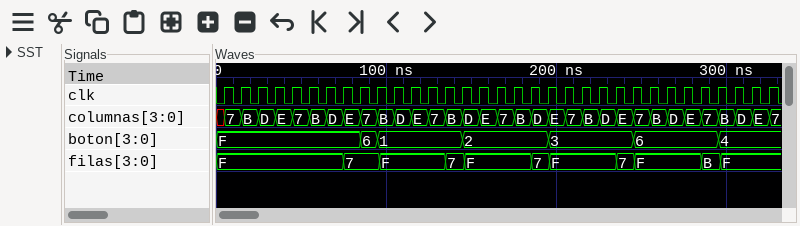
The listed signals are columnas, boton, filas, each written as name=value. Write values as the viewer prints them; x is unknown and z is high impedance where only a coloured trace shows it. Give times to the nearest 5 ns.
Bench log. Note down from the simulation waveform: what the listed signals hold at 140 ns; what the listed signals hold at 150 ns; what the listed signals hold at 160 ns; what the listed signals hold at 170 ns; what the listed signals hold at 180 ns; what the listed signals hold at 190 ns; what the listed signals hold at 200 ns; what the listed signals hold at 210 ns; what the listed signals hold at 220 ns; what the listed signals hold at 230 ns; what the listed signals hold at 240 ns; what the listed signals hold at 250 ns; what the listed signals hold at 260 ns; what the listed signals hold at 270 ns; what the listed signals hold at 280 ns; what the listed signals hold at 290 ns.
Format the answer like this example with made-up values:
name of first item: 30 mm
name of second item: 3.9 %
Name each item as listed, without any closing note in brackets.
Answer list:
what the listed signals hold at 140 ns: columnas=B, boton=1, filas=7
what the listed signals hold at 150 ns: columnas=D, boton=2, filas=F
what the listed signals hold at 160 ns: columnas=E, boton=2, filas=F
what the listed signals hold at 170 ns: columnas=7, boton=2, filas=F
what the listed signals hold at 180 ns: columnas=B, boton=2, filas=F
what the listed signals hold at 190 ns: columnas=D, boton=2, filas=7
what the listed signals hold at 200 ns: columnas=E, boton=3, filas=F
what the listed signals hold at 210 ns: columnas=7, boton=3, filas=F
what the listed signals hold at 220 ns: columnas=B, boton=3, filas=F
what the listed signals hold at 230 ns: columnas=D, boton=3, filas=F
what the listed signals hold at 240 ns: columnas=E, boton=3, filas=7
what the listed signals hold at 250 ns: columnas=7, boton=6, filas=F
what the listed signals hold at 260 ns: columnas=B, boton=6, filas=F
what the listed signals hold at 270 ns: columnas=D, boton=6, filas=F
what the listed signals hold at 280 ns: columnas=E, boton=6, filas=F
what the listed signals hold at 290 ns: columnas=7, boton=6, filas=B
